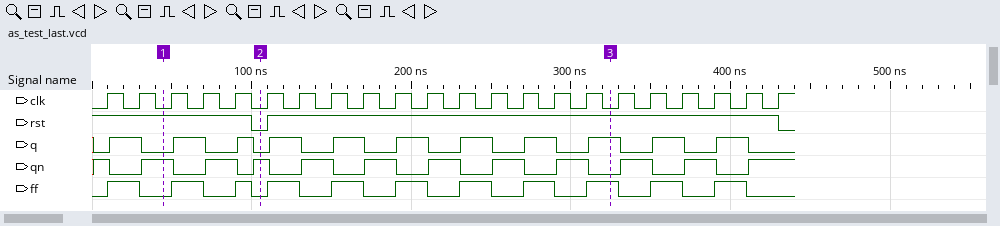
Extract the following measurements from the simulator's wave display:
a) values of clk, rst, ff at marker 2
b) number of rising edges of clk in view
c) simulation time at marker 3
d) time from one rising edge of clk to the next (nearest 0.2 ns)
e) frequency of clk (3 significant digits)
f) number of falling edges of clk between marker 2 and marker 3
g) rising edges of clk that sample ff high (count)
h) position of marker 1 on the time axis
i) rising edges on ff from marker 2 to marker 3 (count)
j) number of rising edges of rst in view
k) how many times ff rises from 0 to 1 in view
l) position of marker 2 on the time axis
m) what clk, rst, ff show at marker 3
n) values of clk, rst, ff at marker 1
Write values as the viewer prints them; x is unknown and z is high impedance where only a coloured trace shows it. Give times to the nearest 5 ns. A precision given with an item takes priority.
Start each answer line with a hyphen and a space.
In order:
- clk=0, rst=0, ff=0
- 22
- 325 ns
- 20 ns
- 50.0 MHz
- 11
- 10
- 45 ns
- 6
- 1
- 11
- 105 ns
- clk=0, rst=1, ff=1
- clk=0, rst=1, ff=0
